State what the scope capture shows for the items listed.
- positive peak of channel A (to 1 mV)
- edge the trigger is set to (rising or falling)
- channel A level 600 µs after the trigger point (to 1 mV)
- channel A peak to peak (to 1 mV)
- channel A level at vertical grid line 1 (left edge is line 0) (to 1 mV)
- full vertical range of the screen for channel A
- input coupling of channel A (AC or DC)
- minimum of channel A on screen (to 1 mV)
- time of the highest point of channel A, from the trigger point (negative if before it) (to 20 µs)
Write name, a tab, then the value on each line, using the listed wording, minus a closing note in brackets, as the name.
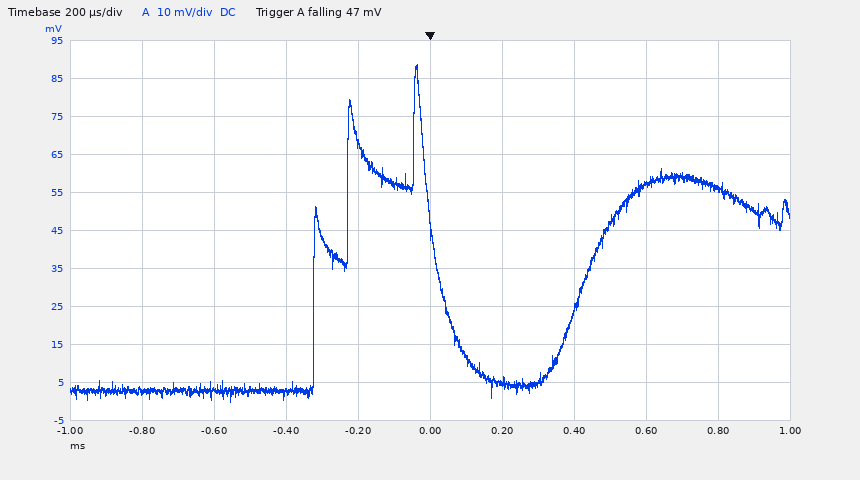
positive peak of channel A	89 mV
edge the trigger is set to	falling
channel A level 600 µs after the trigger point	57 mV
channel A peak to peak	89 mV
channel A level at vertical grid line 1 (left edge is line 0)	3 mV
full vertical range of the screen for channel A	100 mV
input coupling of channel A	DC
minimum of channel A on screen	0 mV
time of the highest point of channel A, from the trigger point (negative if before it)	-40 µs
